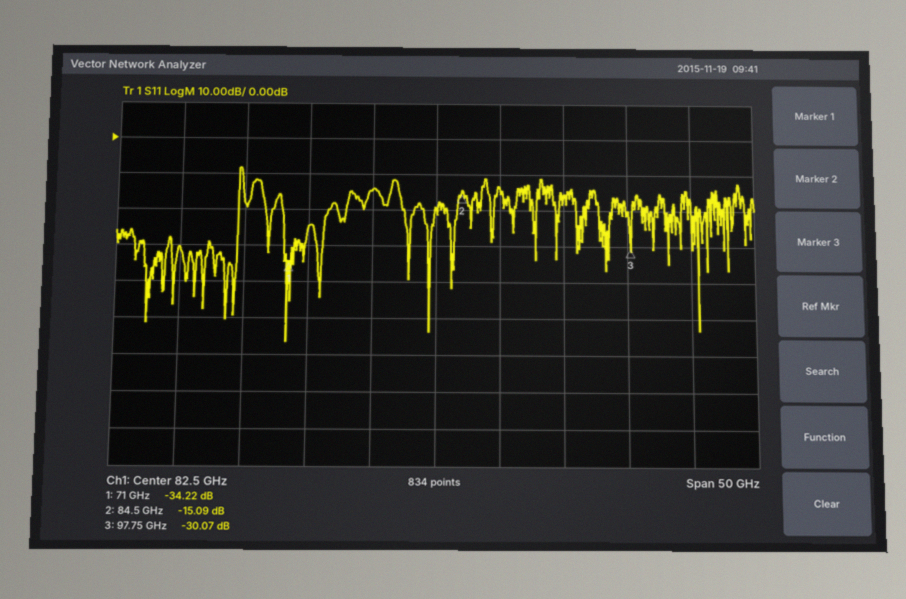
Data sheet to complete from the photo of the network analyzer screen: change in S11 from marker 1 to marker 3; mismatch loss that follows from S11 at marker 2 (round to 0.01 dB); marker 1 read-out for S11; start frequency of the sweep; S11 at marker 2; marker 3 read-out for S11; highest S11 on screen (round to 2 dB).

4.15 dB
0.14 dB
-34.22 dB
57.5 GHz
-15.09 dB
-30.07 dB
-8 dB
